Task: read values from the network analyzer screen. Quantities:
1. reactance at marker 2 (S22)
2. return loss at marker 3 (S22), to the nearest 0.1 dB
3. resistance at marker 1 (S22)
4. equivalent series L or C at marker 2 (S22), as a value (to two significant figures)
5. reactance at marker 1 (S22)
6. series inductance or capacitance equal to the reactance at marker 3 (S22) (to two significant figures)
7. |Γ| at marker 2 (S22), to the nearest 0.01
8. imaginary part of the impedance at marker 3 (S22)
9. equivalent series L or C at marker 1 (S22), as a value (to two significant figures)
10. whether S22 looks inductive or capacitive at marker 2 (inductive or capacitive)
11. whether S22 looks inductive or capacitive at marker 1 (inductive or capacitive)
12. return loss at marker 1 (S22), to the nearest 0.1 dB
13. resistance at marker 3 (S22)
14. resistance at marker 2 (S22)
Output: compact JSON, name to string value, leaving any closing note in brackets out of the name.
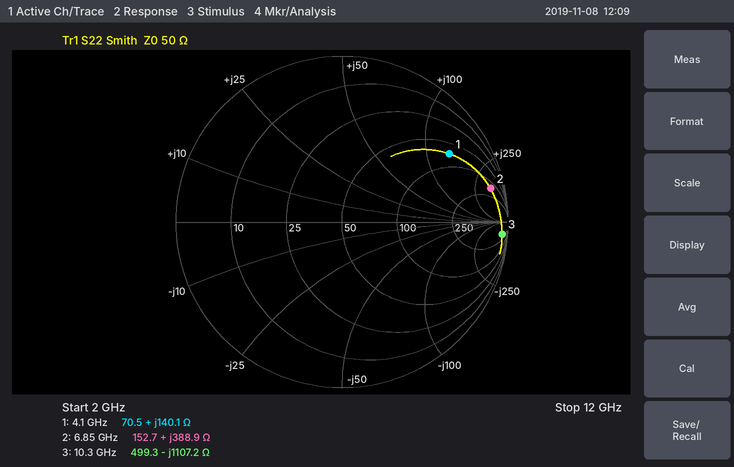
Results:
{"reactance at marker 2": "+388.9 Ω", "return loss at marker 3 (S22), to the nearest 0.1 dB": "0.3 dB", "resistance at marker 1": "70.5 Ω", "equivalent series L or C at marker 2 (S22), as a value": "9.0 nH", "reactance at marker 1": "+140.1 Ω", "series inductance or capacitance equal to the reactance at marker 3 (S22)": "14 fF", "|Γ| at marker 2 (S22), to the nearest 0.01": "0.92", "imaginary part of the impedance at marker 3": "-1107.2 Ω", "equivalent series L or C at marker 1 (S22), as a value": "5.4 nH", "whether S22 looks inductive or capacitive at marker 2": "inductive", "whether S22 looks inductive or capacitive at marker 1": "inductive", "return loss at marker 1 (S22), to the nearest 0.1 dB": "2.3 dB", "resistance at marker 3": "499.3 Ω", "resistance at marker 2": "152.7 Ω"}
